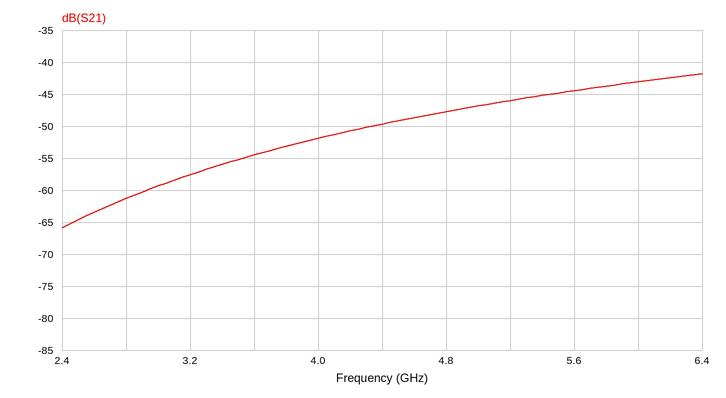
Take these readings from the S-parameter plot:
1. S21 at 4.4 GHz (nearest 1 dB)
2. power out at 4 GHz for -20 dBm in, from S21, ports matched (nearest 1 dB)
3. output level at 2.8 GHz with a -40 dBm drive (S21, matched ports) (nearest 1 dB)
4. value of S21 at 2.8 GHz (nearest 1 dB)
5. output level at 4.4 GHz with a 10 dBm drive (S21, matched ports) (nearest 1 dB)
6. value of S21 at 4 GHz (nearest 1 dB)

-50 dB
-72 dBm
-101 dBm
-61 dB
-40 dBm
-52 dB
